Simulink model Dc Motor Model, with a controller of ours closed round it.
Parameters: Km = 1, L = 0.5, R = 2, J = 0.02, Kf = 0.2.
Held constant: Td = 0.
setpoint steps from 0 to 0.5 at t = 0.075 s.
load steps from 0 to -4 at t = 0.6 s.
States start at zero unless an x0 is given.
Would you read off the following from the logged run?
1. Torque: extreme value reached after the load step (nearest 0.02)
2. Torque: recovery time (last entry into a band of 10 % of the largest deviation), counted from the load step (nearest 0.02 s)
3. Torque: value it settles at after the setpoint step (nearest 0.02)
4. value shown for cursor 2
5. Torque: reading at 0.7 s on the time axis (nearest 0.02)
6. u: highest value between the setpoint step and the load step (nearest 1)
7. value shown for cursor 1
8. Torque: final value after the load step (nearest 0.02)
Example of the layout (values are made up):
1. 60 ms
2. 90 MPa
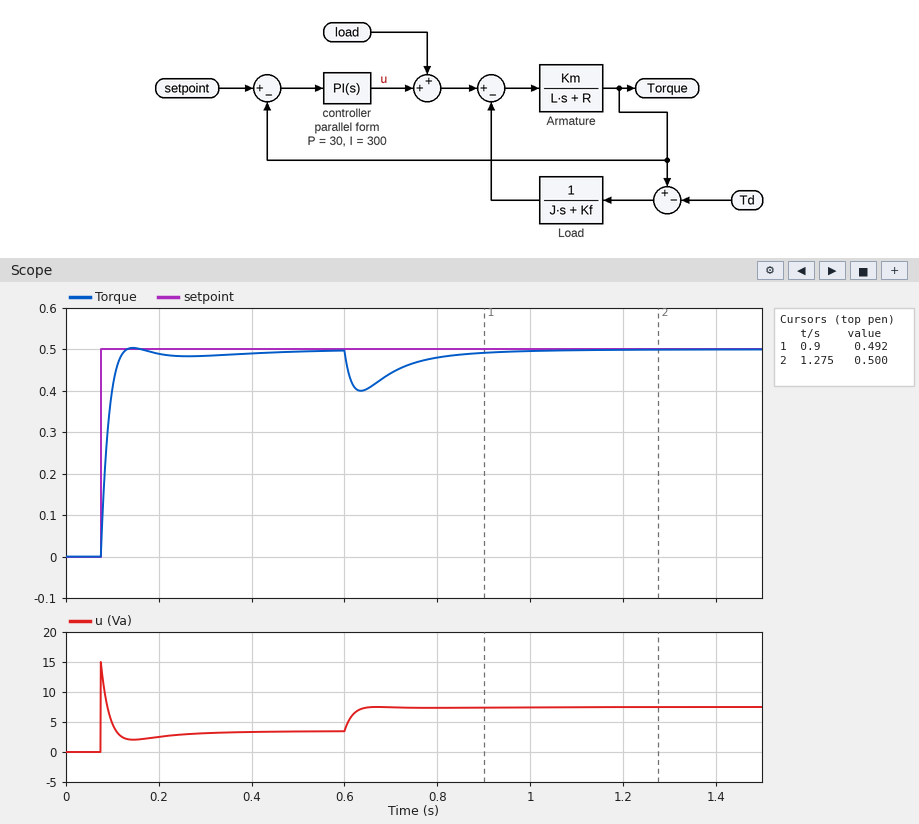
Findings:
1. 0.40
2. 0.28 s
3. 0.50
4. 0.500
5. 0.44
6. 15
7. 0.492
8. 0.50
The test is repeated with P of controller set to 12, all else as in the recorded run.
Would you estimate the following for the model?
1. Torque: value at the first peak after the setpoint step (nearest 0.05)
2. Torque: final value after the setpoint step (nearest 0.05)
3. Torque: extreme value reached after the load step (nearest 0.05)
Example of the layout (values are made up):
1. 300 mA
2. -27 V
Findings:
1. 0.55
2. 0.50
3. 0.35
